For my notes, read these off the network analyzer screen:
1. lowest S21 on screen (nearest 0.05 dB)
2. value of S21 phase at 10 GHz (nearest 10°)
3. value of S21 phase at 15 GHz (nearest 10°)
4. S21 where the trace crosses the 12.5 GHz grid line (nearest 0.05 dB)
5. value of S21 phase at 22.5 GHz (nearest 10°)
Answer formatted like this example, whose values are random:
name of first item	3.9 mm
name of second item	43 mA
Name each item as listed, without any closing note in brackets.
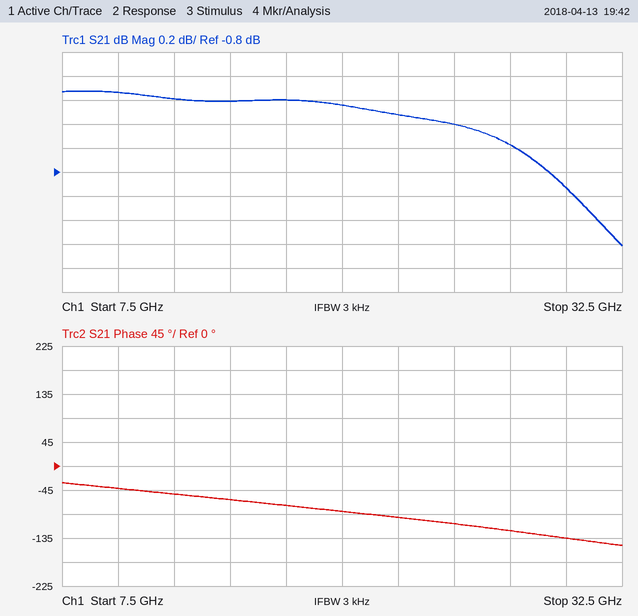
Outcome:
lowest S21 on screen	-1.40 dB
value of S21 phase at 10 GHz	-40°
value of S21 phase at 15 GHz	-60°
S21 where the trace crosses the 12.5 GHz grid line	-0.20 dB
value of S21 phase at 22.5 GHz	-100°
